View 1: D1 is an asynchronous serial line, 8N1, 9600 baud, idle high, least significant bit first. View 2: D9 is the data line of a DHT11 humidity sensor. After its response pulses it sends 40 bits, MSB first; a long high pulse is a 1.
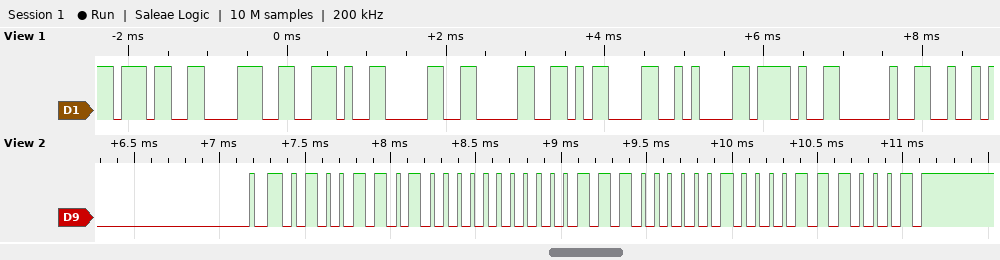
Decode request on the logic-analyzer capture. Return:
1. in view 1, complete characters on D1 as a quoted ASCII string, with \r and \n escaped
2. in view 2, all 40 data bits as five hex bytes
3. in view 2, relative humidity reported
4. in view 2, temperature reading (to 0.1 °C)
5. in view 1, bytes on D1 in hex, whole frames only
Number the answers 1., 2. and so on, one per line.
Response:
1. "78.00\r\n/ "
2. 4D 00 1C 08 71
3. 77 %
4. 28.8 °C
5. 0x37 0x38 0x2E 0x30 0x30 0x0D 0x0A 0x2F 0x20
